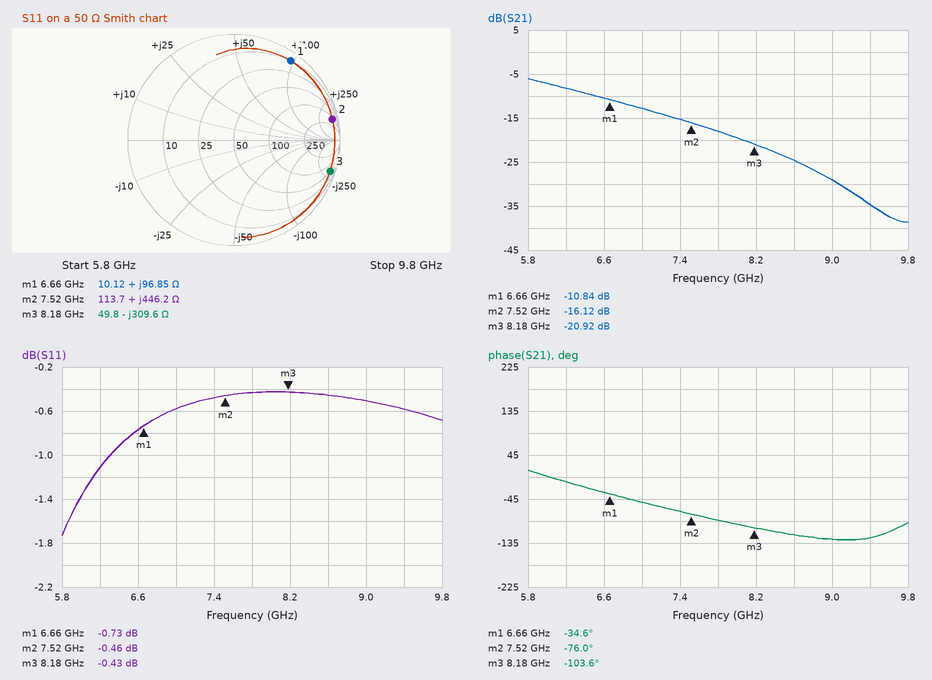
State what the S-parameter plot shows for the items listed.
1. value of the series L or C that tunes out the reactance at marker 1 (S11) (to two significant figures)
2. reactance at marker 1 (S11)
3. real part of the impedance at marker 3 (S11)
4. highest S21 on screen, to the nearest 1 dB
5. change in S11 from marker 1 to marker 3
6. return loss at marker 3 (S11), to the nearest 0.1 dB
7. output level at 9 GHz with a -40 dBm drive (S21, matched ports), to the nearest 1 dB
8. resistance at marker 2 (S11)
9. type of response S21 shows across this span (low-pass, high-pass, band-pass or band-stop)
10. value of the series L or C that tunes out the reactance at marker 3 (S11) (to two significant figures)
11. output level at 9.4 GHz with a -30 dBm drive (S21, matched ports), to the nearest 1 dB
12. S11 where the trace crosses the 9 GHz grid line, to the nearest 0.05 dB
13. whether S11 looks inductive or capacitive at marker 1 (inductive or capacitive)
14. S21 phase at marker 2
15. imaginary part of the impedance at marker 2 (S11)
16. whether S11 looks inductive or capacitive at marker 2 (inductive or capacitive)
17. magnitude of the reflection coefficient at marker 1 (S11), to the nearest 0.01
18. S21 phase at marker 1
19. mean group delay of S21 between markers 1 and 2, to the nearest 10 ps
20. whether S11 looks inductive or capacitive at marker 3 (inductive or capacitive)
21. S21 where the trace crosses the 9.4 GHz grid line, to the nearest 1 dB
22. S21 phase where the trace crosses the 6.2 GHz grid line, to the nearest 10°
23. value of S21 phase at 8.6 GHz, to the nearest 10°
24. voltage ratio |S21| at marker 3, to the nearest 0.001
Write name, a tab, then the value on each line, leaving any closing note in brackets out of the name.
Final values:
value of the series L or C that tunes out the reactance at marker 1 (S11)	250 fF
reactance at marker 1	+96.85 Ω
real part of the impedance at marker 3	49.8 Ω
highest S21 on screen, to the nearest 1 dB	-6 dB
change in S11 from marker 1 to marker 3	0.30 dB
return loss at marker 3 (S11), to the nearest 0.1 dB	0.4 dB
output level at 9 GHz with a -40 dBm drive (S21, matched ports), to the nearest 1 dB	-69 dBm
resistance at marker 2	113.7 Ω
type of response S21 shows across this span	low-pass
value of the series L or C that tunes out the reactance at marker 3 (S11)	6.0 nH
output level at 9.4 GHz with a -30 dBm drive (S21, matched ports), to the nearest 1 dB	-65 dBm
S11 where the trace crosses the 9 GHz grid line, to the nearest 0.05 dB	-0.50 dB
whether S11 looks inductive or capacitive at marker 1	inductive
S21 phase at marker 2	-76.0°
imaginary part of the impedance at marker 2	+446.2 Ω
whether S11 looks inductive or capacitive at marker 2	inductive
magnitude of the reflection coefficient at marker 1 (S11), to the nearest 0.01	0.92
S21 phase at marker 1	-34.6°
mean group delay of S21 between markers 1 and 2, to the nearest 10 ps	130 ps
whether S11 looks inductive or capacitive at marker 3	capacitive
S21 where the trace crosses the 9.4 GHz grid line, to the nearest 1 dB	-35 dB
S21 phase where the trace crosses the 6.2 GHz grid line, to the nearest 10°	-10°
value of S21 phase at 8.6 GHz, to the nearest 10°	-120°
voltage ratio |S21| at marker 3, to the nearest 0.001	0.090
